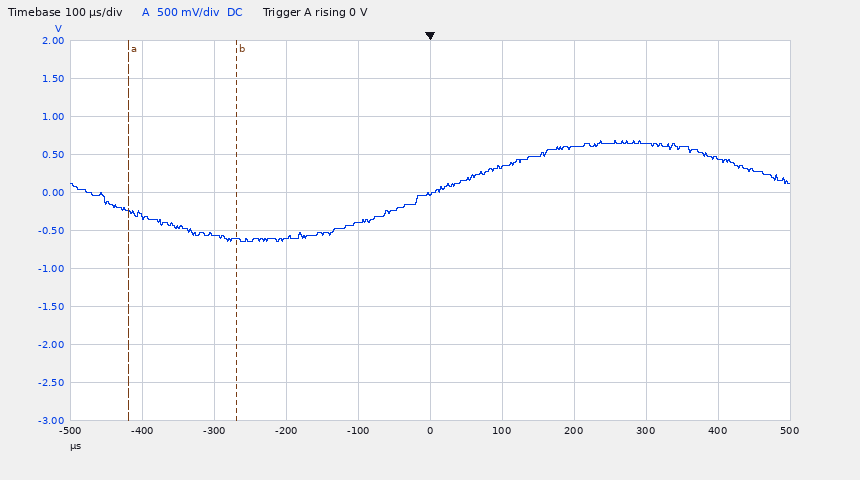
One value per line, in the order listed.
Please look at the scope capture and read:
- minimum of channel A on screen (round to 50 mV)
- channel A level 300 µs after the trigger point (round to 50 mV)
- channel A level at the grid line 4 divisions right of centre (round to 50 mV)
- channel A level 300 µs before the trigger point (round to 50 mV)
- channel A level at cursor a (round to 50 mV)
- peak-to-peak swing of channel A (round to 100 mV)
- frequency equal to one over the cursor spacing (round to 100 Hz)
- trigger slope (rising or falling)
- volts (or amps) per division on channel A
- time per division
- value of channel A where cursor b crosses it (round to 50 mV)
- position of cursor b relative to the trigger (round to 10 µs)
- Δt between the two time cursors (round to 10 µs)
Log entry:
-650 mV
650 mV
450 mV
-550 mV
-250 mV
1.30 V
6.7 kHz
rising
500 mV
100 µs
-600 mV
-270 µs
150 µs
